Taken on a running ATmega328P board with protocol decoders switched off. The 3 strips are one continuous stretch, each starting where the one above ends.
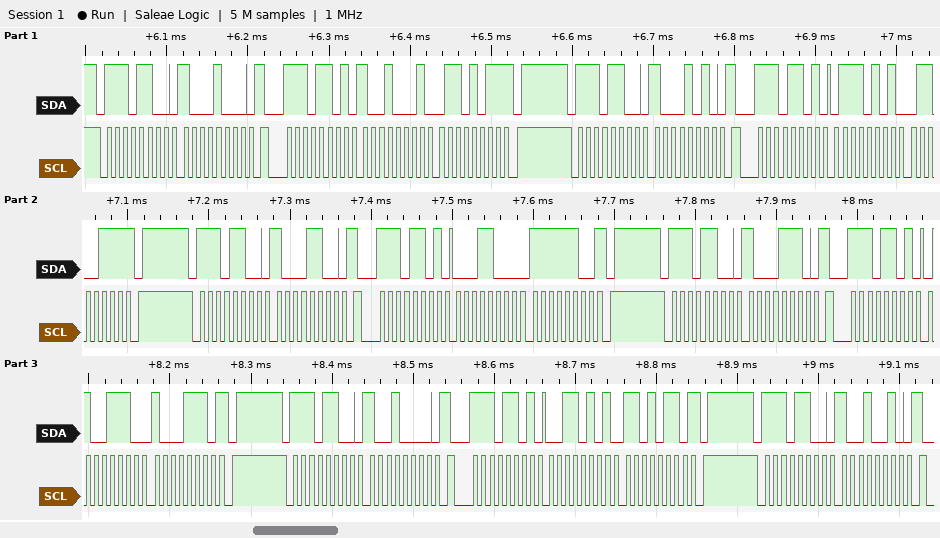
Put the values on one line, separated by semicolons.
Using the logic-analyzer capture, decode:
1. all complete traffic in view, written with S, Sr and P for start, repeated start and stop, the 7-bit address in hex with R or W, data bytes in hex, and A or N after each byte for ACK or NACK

S 76W A 88 A Sr 76R A 91 A 6B N P S 76W A 8A A Sr 76R A 75 A 67 N P S 76W A 8C A Sr 76R A 18 A FC N P S 76W A 8E A Sr 76R A 4E A 8E N P S 76W A 90 A Sr 76R A 35 A D6 N P S 76W A 92 A
